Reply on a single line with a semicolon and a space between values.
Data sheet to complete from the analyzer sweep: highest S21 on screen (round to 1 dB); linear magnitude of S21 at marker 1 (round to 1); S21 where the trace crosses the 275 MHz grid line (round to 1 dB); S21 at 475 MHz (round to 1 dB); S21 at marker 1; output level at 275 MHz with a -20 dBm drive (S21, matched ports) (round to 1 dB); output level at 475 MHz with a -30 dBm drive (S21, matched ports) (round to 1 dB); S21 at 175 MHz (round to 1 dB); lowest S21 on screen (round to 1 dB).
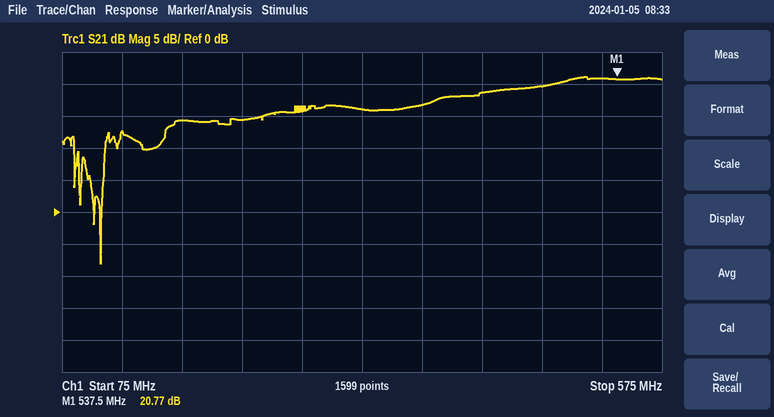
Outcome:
21 dB; 11; 16 dB; 20 dB; 20.77 dB; -4 dBm; -10 dBm; 14 dB; -8 dB
